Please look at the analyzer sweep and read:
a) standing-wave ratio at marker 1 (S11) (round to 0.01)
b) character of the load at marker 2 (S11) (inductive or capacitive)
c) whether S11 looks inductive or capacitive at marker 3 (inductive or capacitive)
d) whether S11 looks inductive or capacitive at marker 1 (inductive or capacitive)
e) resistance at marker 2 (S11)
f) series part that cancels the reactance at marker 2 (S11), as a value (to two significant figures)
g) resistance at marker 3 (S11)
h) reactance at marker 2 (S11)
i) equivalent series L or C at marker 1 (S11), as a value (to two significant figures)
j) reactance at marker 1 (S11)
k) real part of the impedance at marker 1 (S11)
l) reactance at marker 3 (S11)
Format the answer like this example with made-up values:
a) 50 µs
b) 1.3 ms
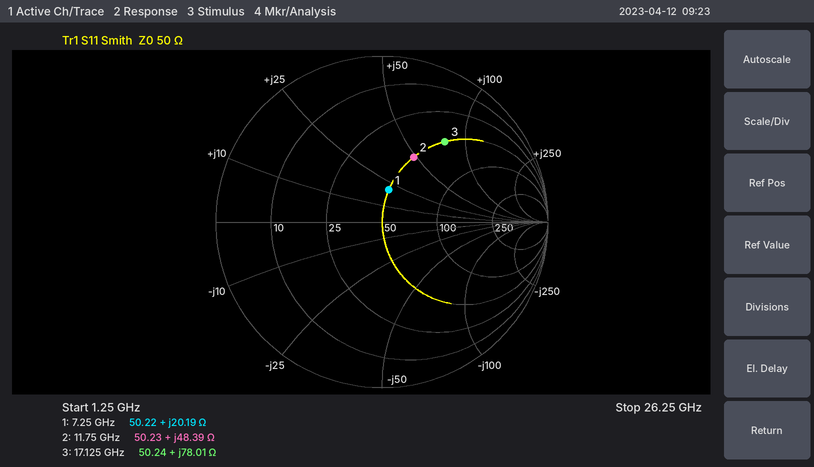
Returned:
a) 1.49
b) inductive
c) inductive
d) inductive
e) 50.23 Ω
f) 280 fF
g) 50.24 Ω
h) +48.39 Ω
i) 440 pH
j) +20.19 Ω
k) 50.22 Ω
l) +78.01 Ω
